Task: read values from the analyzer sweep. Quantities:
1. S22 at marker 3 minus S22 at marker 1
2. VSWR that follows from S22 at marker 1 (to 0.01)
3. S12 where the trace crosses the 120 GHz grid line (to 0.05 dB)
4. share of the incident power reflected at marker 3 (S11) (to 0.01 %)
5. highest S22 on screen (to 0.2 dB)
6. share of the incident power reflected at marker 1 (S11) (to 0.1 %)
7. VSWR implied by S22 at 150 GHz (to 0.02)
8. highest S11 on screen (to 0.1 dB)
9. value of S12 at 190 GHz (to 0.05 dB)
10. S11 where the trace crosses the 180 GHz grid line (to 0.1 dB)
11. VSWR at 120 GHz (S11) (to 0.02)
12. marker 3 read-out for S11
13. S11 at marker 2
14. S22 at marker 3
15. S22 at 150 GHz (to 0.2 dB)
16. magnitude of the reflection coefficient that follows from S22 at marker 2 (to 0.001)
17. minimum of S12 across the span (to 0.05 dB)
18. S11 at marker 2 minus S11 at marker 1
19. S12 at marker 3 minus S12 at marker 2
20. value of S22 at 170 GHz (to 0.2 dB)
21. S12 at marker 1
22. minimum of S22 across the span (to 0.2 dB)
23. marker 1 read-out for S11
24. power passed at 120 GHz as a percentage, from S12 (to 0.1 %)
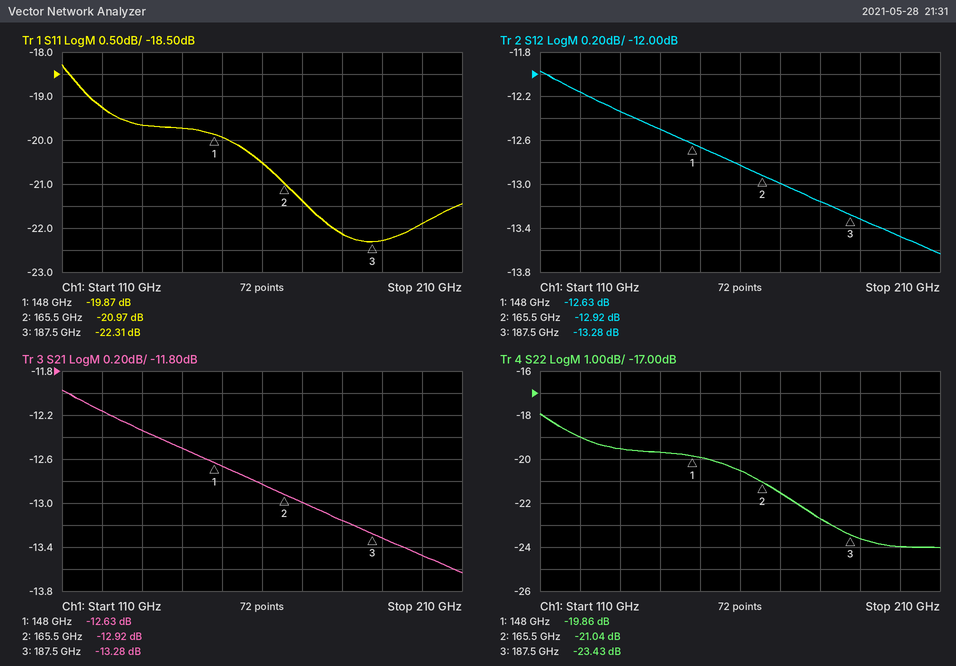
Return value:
-3.57 dB
1.23
-12.15 dB
0.59 %
-18.0 dB
1.0 %
1.22
-18.3 dB
-13.30 dB
-22.1 dB
1.24
-22.31 dB
-20.97 dB
-23.43 dB
-20.0 dB
0.089
-13.65 dB
-1.10 dB
-0.36 dB
-21.6 dB
-12.63 dB
-24.0 dB
-19.87 dB
6.1 %
